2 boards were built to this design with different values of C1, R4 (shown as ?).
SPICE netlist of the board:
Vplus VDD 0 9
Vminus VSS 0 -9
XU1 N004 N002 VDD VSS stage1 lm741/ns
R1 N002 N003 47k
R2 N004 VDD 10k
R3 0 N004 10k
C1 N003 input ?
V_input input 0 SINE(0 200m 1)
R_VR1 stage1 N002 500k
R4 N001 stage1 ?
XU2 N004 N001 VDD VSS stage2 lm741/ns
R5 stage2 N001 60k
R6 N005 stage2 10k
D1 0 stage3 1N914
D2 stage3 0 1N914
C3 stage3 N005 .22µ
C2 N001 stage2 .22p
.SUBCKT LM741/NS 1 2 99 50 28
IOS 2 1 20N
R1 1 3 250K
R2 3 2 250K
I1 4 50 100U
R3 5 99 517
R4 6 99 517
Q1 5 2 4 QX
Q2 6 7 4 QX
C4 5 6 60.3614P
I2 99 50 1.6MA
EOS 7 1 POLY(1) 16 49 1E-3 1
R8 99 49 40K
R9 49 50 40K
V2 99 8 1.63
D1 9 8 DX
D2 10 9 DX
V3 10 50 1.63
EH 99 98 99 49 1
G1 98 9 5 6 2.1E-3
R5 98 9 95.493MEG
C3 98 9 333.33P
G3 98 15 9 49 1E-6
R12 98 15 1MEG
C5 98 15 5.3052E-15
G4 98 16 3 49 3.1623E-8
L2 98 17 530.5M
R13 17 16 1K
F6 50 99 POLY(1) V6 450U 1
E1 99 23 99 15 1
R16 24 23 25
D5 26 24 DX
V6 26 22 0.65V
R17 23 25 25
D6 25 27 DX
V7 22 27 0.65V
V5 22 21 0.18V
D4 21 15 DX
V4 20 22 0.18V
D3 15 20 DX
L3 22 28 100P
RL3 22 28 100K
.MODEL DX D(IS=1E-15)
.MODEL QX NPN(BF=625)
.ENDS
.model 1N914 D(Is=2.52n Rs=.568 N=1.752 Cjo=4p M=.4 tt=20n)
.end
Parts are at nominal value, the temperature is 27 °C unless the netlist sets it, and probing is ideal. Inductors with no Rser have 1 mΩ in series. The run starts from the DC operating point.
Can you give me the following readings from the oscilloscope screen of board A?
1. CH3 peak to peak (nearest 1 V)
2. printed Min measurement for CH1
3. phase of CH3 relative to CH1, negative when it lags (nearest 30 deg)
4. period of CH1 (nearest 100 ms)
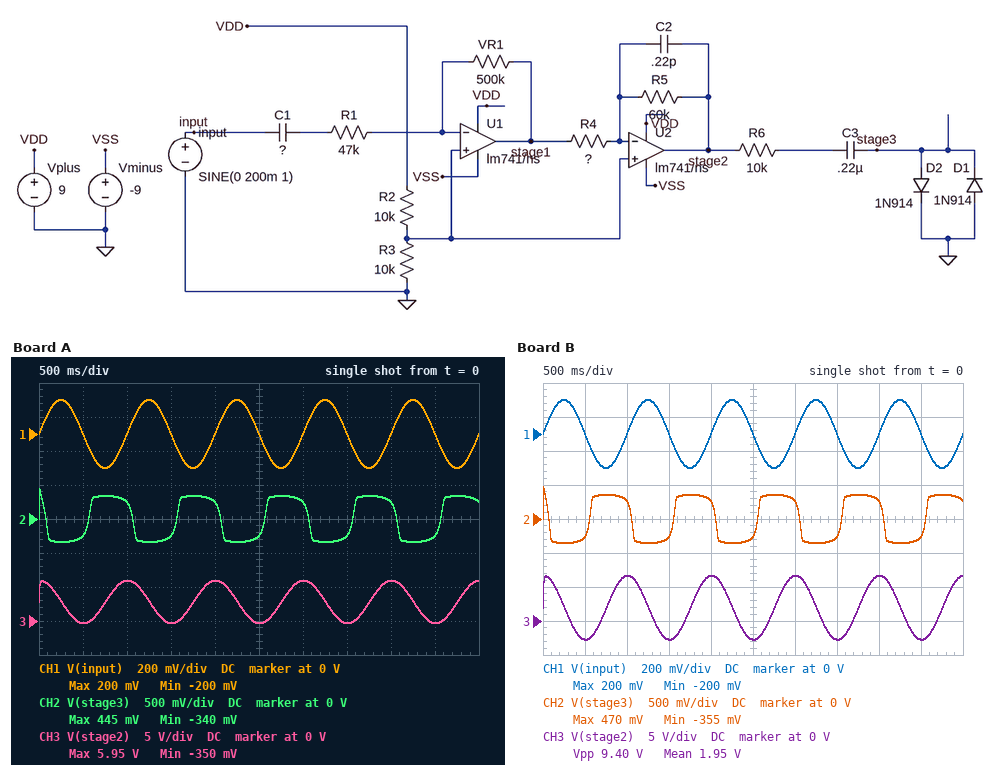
6 V
-200 mV
90 deg
1.0 s
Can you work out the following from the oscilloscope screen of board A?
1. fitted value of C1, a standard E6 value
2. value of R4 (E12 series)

150 nF
1.8 kΩ
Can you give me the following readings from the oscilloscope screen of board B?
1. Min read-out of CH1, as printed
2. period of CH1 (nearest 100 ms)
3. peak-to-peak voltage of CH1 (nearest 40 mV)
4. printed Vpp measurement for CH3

-200 mV
1.0 s
400 mV
9.40 V
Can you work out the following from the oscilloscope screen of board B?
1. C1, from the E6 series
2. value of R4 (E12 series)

150 nF
1.2 kΩ
